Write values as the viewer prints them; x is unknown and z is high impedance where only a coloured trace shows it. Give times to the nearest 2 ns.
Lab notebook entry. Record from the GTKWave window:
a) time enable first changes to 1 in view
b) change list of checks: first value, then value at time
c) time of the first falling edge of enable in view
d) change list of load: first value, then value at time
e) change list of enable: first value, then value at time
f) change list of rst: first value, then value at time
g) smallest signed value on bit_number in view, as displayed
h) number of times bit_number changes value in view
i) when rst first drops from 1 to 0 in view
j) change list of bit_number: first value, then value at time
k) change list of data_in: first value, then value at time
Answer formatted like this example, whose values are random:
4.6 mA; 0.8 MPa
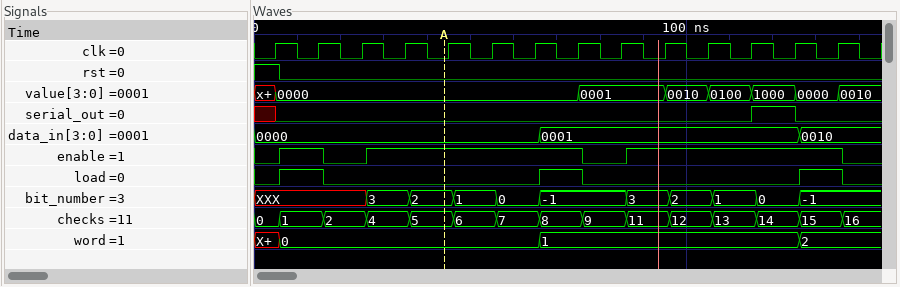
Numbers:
6 ns; 0, 1 at 6 ns, 2 at 16 ns, 4 at 26 ns, 5 at 36 ns, 6 at 46 ns, 7 at 56 ns, 8 at 66 ns, 9 at 76 ns, 11 at 86 ns, 12 at 96 ns, 13 at 106 ns, 14 at 116 ns, 15 at 126 ns, 16 at 136 ns; 16 ns; 0, 1 at 6 ns, 0 at 16 ns, 1 at 66 ns, 0 at 76 ns, 1 at 126 ns, 0 at 136 ns; 0, 1 at 6 ns, 0 at 16 ns, 1 at 26 ns, 0 at 76 ns, 1 at 86 ns, 0 at 136 ns; 1, 0 at 6 ns; -1; 10; 6 ns; XXX, 3 at 26 ns, 2 at 36 ns, 1 at 46 ns, 0 at 56 ns, -1 at 66 ns, 3 at 86 ns, 2 at 96 ns, 1 at 106 ns, 0 at 116 ns, -1 at 126 ns; 0000, 0001 at 66 ns, 0010 at 126 ns
